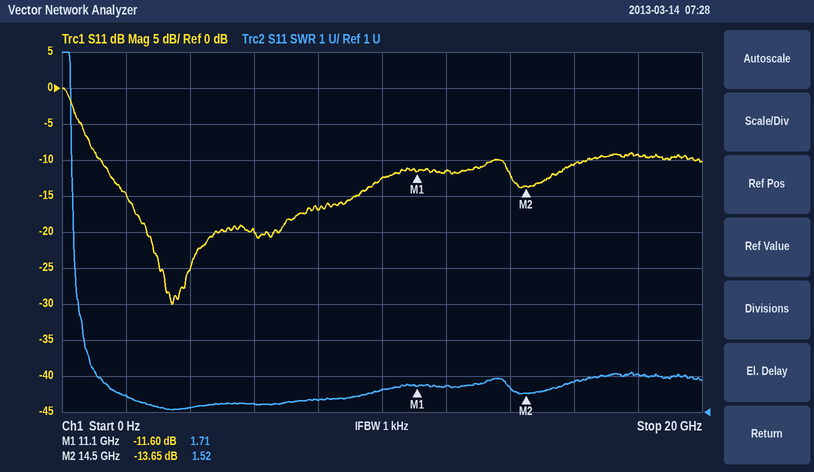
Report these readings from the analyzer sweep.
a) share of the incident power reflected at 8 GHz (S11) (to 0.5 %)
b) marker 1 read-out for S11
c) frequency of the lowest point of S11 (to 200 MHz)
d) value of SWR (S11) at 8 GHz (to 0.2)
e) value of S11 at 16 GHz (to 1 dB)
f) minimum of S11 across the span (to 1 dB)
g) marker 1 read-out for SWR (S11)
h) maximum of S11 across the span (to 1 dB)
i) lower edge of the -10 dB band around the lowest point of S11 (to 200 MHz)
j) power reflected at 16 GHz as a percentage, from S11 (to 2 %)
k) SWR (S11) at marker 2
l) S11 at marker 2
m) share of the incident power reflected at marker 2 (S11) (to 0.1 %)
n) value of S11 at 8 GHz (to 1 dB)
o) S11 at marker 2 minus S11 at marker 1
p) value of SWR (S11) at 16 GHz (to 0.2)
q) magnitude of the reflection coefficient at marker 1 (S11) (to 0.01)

2.0 %
-11.60 dB
3.4 GHz
1.4
-11 dB
-30 dB
1.71
0 dB
1.2 GHz
8 %
1.52
-13.65 dB
4.3 %
-17 dB
-2.05 dB
1.8
0.26
